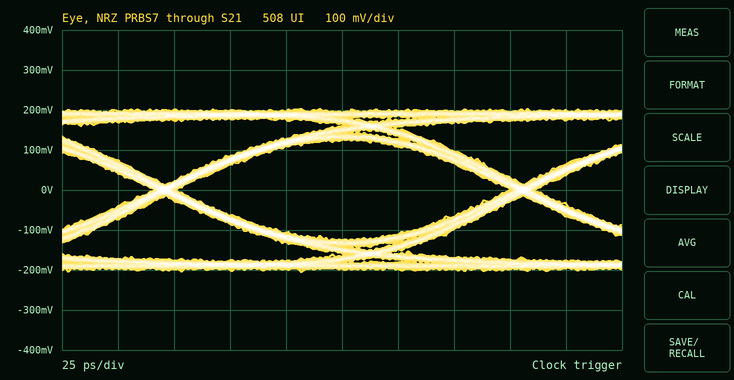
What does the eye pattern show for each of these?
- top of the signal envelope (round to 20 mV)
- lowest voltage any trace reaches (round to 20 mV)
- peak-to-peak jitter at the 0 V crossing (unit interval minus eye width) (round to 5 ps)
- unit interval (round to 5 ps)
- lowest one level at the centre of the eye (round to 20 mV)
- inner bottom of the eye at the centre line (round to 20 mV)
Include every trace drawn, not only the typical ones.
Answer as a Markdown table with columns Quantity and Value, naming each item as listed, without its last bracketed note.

| Quantity | Value |
|---|---|
| top of the signal envelope | 200 mV |
| lowest voltage any trace reaches | -200 mV |
| peak-to-peak jitter at the 0 V crossing (unit interval minus eye width) | 10 ps |
| unit interval | 160 ps |
| lowest one level at the centre of the eye | 120 mV |
| inner bottom of the eye at the centre line | -120 mV |
